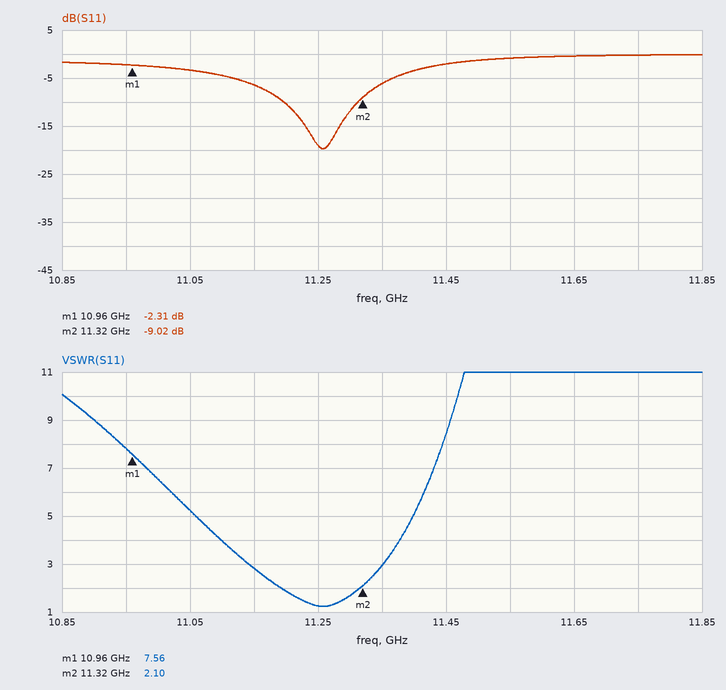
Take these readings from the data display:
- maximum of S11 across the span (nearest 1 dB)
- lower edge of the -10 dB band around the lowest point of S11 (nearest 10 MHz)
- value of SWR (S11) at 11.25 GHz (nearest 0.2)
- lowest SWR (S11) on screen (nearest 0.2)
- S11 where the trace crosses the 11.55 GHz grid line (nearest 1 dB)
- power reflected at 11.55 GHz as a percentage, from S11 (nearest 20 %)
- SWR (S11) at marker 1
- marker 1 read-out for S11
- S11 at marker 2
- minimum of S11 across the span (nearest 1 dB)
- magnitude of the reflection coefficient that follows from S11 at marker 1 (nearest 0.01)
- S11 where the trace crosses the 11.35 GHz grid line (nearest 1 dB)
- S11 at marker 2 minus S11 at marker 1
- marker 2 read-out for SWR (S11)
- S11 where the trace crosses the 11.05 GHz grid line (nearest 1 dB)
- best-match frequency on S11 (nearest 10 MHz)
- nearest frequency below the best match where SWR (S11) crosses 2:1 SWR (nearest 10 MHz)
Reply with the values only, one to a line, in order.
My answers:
0 dB
11.20 GHz
1.2
1.2
-1 dB
80 %
7.56
-2.31 dB
-9.02 dB
-20 dB
0.77
-6 dB
-6.71 dB
2.10
-3 dB
11.26 GHz
11.19 GHz
